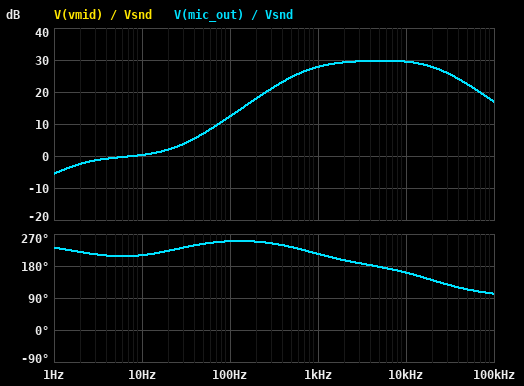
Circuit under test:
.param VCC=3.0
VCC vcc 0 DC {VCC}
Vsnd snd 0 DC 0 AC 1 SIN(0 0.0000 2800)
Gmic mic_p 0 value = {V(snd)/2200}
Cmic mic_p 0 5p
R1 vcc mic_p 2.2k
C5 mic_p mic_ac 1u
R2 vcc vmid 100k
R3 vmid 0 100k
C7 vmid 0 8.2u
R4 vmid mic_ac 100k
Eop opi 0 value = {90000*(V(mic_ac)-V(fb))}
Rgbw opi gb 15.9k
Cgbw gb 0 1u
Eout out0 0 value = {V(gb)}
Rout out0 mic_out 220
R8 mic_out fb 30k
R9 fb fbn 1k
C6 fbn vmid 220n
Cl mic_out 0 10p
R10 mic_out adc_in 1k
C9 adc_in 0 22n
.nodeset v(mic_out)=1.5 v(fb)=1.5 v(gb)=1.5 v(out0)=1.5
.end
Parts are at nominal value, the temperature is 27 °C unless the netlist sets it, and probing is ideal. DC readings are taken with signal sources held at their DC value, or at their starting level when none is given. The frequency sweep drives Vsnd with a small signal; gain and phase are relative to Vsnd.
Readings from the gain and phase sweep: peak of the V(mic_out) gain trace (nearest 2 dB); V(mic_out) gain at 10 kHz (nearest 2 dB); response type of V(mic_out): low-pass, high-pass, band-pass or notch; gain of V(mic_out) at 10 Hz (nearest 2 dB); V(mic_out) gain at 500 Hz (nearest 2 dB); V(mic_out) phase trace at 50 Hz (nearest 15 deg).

30 dB
30 dB
band-pass
0 dB
24 dB
240 deg
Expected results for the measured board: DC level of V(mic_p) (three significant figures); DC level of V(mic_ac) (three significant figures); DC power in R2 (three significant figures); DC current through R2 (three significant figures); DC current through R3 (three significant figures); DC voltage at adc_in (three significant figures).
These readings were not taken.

3.00 V
1.50 V
22.5 µW
15.0 µA
15.0 µA
1.50 V
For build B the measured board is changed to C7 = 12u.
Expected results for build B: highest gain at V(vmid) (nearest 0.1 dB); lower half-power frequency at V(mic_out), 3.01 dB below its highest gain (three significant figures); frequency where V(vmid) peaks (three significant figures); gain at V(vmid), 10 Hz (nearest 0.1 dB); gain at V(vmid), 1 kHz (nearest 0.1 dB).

-23.5 dB
741 Hz
649 mHz
-33.3 dB
-39.4 dB
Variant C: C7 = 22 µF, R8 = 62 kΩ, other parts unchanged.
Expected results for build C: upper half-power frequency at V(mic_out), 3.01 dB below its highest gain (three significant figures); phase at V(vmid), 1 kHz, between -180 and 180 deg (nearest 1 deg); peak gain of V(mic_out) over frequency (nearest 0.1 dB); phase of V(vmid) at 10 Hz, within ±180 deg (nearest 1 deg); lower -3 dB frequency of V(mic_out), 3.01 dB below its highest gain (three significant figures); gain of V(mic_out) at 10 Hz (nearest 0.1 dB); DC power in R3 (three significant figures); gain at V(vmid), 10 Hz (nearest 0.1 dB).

13.4 kHz
123 deg
36.0 dB
154 deg
721 Hz
2.1 dB
22.5 µW
-38.5 dB
